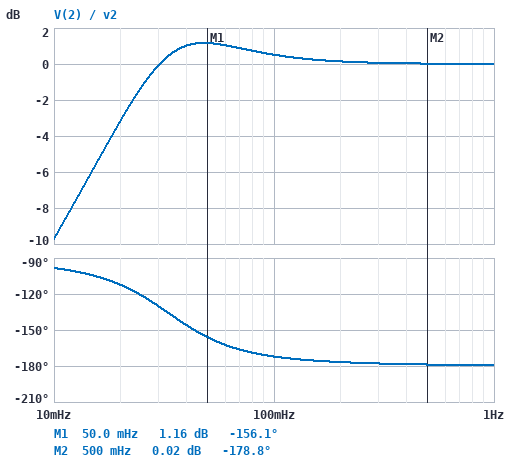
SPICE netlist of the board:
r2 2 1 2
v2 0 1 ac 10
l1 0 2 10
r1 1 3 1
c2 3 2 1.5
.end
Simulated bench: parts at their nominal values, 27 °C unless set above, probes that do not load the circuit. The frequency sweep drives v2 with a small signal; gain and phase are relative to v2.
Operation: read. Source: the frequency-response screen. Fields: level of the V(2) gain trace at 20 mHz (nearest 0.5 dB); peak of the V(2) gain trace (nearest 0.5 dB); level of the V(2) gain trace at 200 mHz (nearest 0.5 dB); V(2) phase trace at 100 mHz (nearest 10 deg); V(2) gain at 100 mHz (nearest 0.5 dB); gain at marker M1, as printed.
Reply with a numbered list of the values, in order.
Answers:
1. -3.0 dB
2. 1.0 dB
3. 0 dB
4. -170 deg
5. 0.5 dB
6. 1.16 dB
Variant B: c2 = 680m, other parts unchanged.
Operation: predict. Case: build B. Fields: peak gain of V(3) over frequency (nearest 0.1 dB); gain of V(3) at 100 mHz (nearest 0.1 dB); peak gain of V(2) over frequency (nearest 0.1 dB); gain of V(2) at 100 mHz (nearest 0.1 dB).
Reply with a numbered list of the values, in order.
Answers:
1. 0 dB
2. -0.6 dB
3. 0.9 dB
4. 0.8 dB
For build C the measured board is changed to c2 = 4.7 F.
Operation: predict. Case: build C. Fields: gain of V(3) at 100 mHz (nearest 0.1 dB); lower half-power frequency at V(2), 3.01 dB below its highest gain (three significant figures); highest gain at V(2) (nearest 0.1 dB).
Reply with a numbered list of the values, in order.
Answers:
1. -0.2 dB
2. 15.1 mHz
3. 1.1 dB
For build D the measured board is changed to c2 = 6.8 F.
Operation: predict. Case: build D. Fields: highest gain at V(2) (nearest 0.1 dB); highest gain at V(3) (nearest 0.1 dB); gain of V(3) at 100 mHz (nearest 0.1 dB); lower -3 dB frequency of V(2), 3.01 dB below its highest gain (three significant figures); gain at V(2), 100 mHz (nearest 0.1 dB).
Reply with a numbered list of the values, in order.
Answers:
1. 0.8 dB
2. 0 dB
3. -0.1 dB
4. 13.0 mHz
5. 0.1 dB
